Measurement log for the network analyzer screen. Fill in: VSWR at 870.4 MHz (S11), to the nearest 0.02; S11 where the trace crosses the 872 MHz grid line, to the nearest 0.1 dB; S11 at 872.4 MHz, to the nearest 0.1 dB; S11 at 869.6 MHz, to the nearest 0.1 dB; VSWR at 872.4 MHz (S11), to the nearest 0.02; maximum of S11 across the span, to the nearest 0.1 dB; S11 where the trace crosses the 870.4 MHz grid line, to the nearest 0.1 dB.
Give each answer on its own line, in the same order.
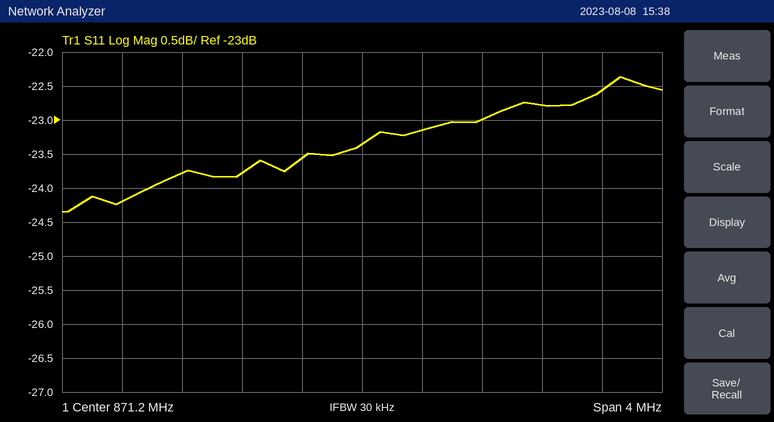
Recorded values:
1.14
-23.0 dB
-22.8 dB
-24.2 dB
1.16
-22.4 dB
-23.8 dB
